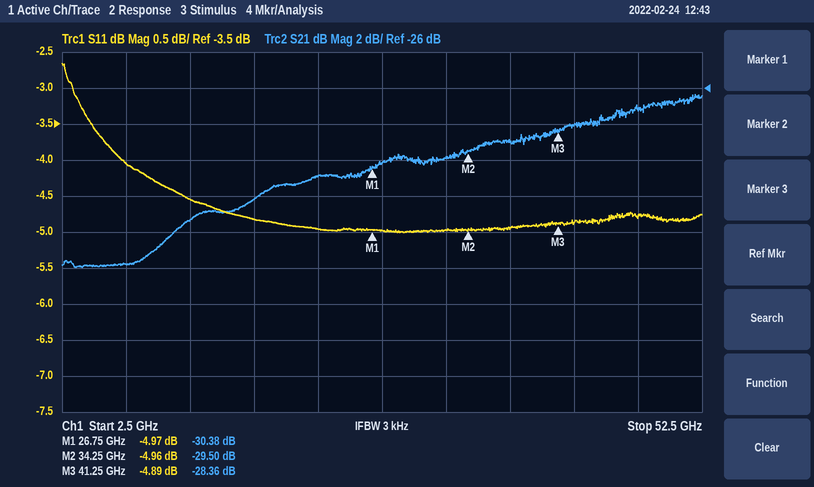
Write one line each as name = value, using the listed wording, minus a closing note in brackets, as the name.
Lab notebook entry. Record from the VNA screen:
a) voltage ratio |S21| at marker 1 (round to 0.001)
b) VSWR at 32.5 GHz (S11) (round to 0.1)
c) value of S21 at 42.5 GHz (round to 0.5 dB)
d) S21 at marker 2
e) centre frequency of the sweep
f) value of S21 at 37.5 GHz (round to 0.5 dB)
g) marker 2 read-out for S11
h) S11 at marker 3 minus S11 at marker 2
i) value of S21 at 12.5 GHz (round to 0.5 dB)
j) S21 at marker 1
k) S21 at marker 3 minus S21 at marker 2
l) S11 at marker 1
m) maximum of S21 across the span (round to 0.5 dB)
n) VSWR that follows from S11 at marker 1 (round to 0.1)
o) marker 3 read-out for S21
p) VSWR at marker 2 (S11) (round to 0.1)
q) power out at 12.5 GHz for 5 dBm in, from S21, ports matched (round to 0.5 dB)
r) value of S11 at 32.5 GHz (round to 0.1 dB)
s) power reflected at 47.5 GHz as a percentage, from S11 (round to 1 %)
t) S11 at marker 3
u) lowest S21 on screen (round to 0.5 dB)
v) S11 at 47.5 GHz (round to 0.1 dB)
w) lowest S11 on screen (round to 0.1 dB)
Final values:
voltage ratio |S21| at marker 1 = 0.030
VSWR at 32.5 GHz (S11) = 3.6
value of S21 at 42.5 GHz = -28.0 dB
S21 at marker 2 = -29.50 dB
centre frequency of the sweep = 27.5 GHz
value of S21 at 37.5 GHz = -29.0 dB
marker 2 read-out for S11 = -4.96 dB
S11 at marker 3 minus S11 at marker 2 = 0.07 dB
value of S21 at 12.5 GHz = -33.5 dB
S21 at marker 1 = -30.38 dB
S21 at marker 3 minus S21 at marker 2 = 1.14 dB
S11 at marker 1 = -4.97 dB
maximum of S21 across the span = -26.5 dB
VSWR that follows from S11 at marker 1 = 3.6
marker 3 read-out for S21 = -28.36 dB
VSWR at marker 2 (S11) = 3.6
power out at 12.5 GHz for 5 dBm in, from S21, ports matched = -28.5 dBm
value of S11 at 32.5 GHz = -5.0 dB
power reflected at 47.5 GHz as a percentage, from S11 = 33 %
S11 at marker 3 = -4.89 dB
lowest S21 on screen = -36.0 dB
S11 at 47.5 GHz = -4.8 dB
lowest S11 on screen = -5.0 dB
